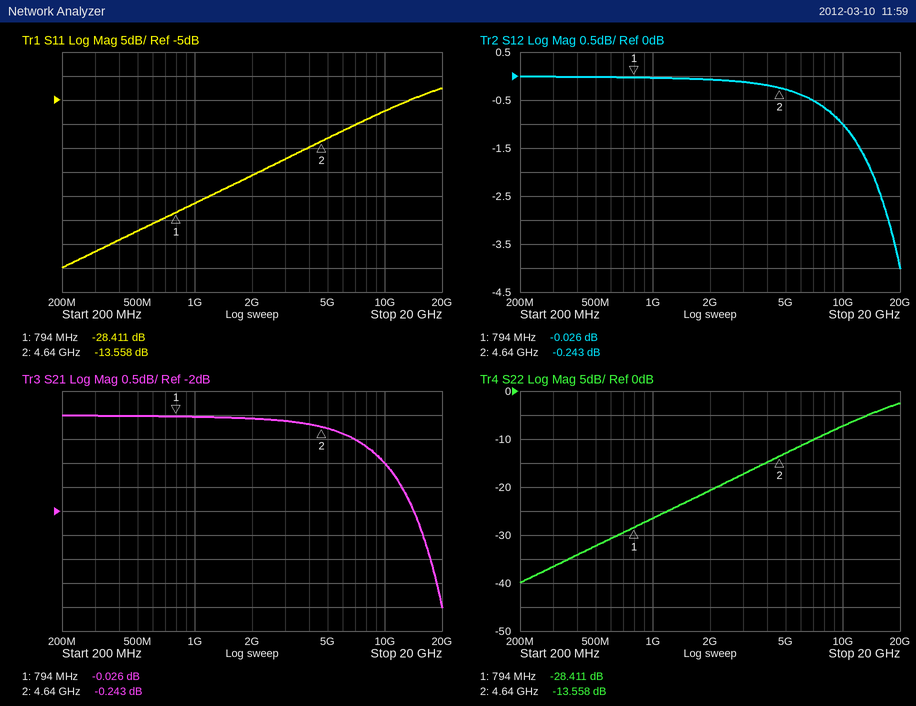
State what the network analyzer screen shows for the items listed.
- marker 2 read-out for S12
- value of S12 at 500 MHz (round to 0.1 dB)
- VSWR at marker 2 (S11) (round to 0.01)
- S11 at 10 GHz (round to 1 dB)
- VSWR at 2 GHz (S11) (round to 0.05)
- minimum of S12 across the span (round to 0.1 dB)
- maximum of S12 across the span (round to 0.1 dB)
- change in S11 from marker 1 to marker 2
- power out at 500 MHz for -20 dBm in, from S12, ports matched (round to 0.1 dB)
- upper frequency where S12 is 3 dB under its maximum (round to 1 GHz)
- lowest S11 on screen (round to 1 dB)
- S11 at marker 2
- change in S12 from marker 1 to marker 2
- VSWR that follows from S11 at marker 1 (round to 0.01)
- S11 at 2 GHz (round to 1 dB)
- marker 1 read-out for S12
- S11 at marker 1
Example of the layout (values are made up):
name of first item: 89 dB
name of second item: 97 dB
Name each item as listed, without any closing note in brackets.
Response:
marker 2 read-out for S12: -0.243 dB
value of S12 at 500 MHz: 0.0 dB
VSWR at marker 2 (S11): 1.53
S11 at 10 GHz: -7 dB
VSWR at 2 GHz (S11): 1.20
minimum of S12 across the span: -4.0 dB
maximum of S12 across the span: 0.0 dB
change in S11 from marker 1 to marker 2: 14.853 dB
power out at 500 MHz for -20 dBm in, from S12, ports matched: -20.0 dBm
upper frequency where S12 is 3 dB under its maximum: 17 GHz
lowest S11 on screen: -40 dB
S11 at marker 2: -13.558 dB
change in S12 from marker 1 to marker 2: -0.217 dB
VSWR that follows from S11 at marker 1: 1.08
S11 at 2 GHz: -21 dB
marker 1 read-out for S12: -0.026 dB
S11 at marker 1: -28.411 dB
